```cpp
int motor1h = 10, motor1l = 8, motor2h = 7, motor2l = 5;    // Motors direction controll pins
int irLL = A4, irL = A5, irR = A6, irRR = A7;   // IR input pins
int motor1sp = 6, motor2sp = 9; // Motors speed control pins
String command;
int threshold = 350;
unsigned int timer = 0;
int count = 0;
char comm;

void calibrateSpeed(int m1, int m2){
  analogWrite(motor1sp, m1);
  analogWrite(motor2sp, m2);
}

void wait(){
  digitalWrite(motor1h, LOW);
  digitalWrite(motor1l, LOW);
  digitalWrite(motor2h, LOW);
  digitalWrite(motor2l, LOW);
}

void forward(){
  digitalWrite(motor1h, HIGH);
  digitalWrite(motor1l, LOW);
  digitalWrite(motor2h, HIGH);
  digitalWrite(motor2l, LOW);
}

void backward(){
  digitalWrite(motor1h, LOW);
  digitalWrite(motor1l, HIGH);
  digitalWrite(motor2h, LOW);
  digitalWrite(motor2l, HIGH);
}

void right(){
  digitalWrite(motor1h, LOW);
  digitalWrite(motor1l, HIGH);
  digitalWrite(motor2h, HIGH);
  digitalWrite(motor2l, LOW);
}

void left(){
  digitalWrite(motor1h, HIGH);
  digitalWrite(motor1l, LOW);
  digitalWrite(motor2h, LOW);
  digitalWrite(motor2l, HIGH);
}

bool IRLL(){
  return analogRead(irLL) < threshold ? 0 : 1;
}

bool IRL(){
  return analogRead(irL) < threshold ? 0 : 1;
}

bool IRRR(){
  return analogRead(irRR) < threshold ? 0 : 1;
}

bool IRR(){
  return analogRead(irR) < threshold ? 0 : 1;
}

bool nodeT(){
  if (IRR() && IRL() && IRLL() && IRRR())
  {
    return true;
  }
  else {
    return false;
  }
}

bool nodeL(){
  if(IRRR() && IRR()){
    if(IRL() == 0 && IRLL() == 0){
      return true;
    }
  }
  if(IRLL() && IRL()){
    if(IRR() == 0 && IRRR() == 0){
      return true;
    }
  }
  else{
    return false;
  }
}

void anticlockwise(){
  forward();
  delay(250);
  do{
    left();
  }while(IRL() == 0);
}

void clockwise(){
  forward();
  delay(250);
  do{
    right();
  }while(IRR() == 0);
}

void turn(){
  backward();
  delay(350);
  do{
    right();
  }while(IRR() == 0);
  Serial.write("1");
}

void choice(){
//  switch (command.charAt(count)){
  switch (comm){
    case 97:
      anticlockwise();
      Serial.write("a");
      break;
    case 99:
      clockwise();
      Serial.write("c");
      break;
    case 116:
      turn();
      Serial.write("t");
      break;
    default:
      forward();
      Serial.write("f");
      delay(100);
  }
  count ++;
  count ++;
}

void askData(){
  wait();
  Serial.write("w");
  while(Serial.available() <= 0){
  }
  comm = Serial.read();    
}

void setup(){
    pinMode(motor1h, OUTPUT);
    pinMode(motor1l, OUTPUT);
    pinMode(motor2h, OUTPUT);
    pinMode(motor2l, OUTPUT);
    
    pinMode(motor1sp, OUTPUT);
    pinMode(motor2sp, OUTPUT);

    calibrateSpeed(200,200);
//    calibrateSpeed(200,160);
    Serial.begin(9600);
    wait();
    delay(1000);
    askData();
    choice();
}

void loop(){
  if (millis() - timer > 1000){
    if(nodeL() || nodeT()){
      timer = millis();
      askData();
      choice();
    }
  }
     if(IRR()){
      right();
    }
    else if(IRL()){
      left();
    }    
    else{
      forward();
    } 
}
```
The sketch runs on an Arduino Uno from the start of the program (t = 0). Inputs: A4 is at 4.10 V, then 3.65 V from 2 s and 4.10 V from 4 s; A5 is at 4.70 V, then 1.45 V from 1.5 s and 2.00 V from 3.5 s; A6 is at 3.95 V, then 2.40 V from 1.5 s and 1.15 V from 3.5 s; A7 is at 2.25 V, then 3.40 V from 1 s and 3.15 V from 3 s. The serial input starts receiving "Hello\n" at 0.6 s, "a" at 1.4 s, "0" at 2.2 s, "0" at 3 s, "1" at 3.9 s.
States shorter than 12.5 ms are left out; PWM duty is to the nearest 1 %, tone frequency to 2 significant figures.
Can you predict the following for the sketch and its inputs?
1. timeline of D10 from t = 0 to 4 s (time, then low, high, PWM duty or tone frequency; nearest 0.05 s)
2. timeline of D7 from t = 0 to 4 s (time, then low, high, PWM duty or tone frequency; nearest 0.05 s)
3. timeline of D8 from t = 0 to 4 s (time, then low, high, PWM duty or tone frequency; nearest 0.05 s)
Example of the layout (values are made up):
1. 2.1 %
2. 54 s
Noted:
1. 0 s low; 1 s high; 1.2 s low; 3.5 s high
2. 0 s low; 1 s high; 3.6 s low
3. 0 s low; 1.2 s high; 3.5 s low
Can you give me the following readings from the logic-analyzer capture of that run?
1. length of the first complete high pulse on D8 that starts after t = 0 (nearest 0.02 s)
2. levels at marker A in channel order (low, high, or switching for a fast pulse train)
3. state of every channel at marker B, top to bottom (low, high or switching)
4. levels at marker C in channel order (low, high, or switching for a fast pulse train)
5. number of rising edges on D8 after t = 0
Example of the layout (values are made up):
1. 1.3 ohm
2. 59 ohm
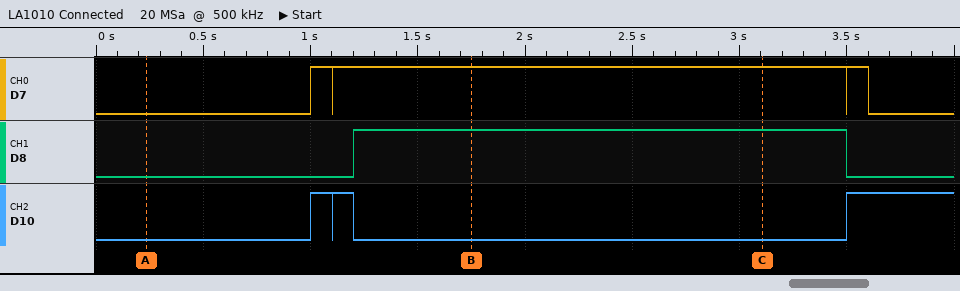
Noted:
1. 2.30 s
2. D7 low, D8 low, D10 low
3. D7 high, D8 high, D10 low
4. D7 high, D8 high, D10 low
5. 1
